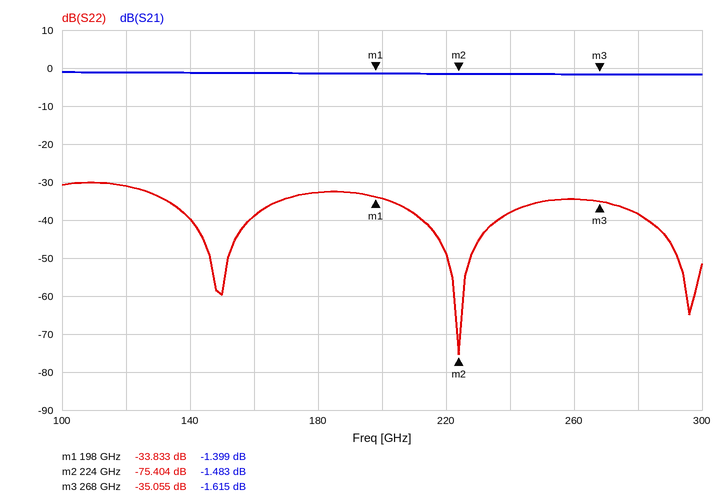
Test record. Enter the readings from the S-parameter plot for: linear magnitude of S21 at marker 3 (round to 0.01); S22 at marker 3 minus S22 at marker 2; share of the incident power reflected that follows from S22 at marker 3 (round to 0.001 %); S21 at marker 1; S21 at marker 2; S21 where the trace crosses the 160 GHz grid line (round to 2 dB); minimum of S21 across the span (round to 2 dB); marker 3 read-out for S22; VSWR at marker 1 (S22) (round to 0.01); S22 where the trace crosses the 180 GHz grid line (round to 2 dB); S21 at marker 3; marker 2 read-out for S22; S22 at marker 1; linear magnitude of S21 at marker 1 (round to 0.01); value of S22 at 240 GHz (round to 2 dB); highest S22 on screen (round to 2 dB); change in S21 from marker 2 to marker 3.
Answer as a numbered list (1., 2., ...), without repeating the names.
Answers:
1. 0.83
2. 40.349 dB
3. 0.031 %
4. -1.399 dB
5. -1.483 dB
6. -2 dB
7. -2 dB
8. -35.055 dB
9. 1.04
10. -32 dB
11. -1.615 dB
12. -75.404 dB
13. -33.833 dB
14. 0.85
15. -38 dB
16. -30 dB
17. -0.132 dB
